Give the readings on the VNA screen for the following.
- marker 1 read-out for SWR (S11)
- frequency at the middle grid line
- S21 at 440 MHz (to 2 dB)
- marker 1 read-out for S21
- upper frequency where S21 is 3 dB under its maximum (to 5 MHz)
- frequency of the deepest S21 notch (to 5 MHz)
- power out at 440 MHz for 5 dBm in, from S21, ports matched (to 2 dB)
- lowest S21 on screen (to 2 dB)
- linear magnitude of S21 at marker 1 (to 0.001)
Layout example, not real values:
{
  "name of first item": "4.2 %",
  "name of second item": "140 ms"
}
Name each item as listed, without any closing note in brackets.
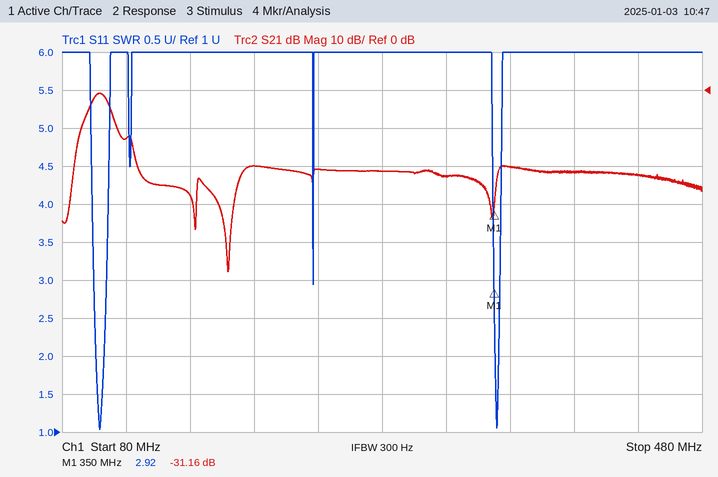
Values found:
{
  "marker 1 read-out for SWR": "2.92",
  "frequency at the middle grid line": "280 MHz",
  "S21 at 440 MHz": "-22 dB",
  "marker 1 read-out for S21": "-31.16 dB",
  "upper frequency where S21 is 3 dB under its maximum": "110 MHz",
  "frequency of the deepest S21 notch": "185 MHz",
  "power out at 440 MHz for 5 dBm in, from S21, ports matched": "-18 dBm",
  "lowest S21 on screen": "-48 dB",
  "linear magnitude of S21 at marker 1": "0.028"
}
